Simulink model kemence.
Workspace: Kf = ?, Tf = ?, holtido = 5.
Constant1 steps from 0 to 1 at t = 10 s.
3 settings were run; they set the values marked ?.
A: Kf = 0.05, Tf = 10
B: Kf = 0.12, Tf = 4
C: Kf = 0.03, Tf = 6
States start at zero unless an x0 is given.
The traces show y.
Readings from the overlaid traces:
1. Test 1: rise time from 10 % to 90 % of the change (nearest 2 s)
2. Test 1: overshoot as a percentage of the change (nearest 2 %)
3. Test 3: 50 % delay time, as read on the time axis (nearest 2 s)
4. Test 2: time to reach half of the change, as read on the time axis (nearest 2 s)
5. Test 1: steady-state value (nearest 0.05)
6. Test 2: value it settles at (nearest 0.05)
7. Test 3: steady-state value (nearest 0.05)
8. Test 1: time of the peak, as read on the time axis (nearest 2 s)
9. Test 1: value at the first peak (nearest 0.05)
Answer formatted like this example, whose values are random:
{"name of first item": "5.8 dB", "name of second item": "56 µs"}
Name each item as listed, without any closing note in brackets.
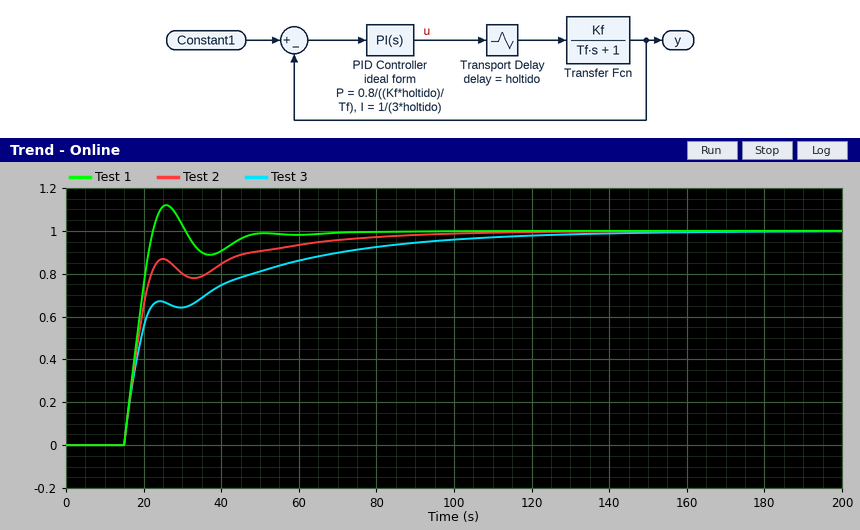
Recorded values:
{"Test 1: rise time from 10 % to 90 % of the change": "6 s", "Test 1: overshoot as a percentage of the change": "12 %", "Test 3: 50 % delay time, as read on the time axis": "20 s", "Test 2: time to reach half of the change, as read on the time axis": "18 s", "Test 1: steady-state value": "1.00", "Test 2: value it settles at": "1.00", "Test 3: steady-state value": "1.00", "Test 1: time of the peak, as read on the time axis": "26 s", "Test 1: value at the first peak": "1.10"}
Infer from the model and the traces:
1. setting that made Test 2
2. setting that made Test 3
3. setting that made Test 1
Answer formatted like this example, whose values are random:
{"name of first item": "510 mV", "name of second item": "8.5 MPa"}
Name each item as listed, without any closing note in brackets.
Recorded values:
{"setting that made Test 2": "C", "setting that made Test 3": "B", "setting that made Test 1": "A"}
